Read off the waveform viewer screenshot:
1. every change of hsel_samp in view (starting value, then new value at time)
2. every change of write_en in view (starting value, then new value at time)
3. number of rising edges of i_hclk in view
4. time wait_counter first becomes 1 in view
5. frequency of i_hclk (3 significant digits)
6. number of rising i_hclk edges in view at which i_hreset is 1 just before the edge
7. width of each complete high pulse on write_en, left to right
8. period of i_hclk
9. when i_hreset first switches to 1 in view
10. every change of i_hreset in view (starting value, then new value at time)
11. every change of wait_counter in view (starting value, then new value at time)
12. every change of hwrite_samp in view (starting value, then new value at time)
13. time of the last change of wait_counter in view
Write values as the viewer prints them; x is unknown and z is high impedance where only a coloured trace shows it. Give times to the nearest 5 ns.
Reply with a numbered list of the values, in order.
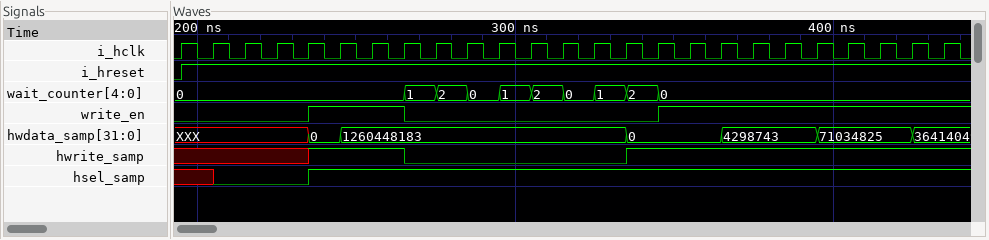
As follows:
1. x, 0 at 205 ns, 1 at 235 ns
2. 0, 1 at 235 ns, 0 at 265 ns, 1 at 345 ns
3. 25
4. 265 ns
5. 100 MHz
6. 24
7. 30 ns
8. 10 ns
9. 195 ns
10. 0, 1 at 195 ns
11. 0, 1 at 265 ns, 2 at 275 ns, 0 at 285 ns, 1 at 295 ns, 2 at 305 ns, 0 at 315 ns, 1 at 325 ns, 2 at 335 ns, 0 at 345 ns
12. x, 1 at 235 ns, 0 at 265 ns, 1 at 335 ns
13. 345 ns
